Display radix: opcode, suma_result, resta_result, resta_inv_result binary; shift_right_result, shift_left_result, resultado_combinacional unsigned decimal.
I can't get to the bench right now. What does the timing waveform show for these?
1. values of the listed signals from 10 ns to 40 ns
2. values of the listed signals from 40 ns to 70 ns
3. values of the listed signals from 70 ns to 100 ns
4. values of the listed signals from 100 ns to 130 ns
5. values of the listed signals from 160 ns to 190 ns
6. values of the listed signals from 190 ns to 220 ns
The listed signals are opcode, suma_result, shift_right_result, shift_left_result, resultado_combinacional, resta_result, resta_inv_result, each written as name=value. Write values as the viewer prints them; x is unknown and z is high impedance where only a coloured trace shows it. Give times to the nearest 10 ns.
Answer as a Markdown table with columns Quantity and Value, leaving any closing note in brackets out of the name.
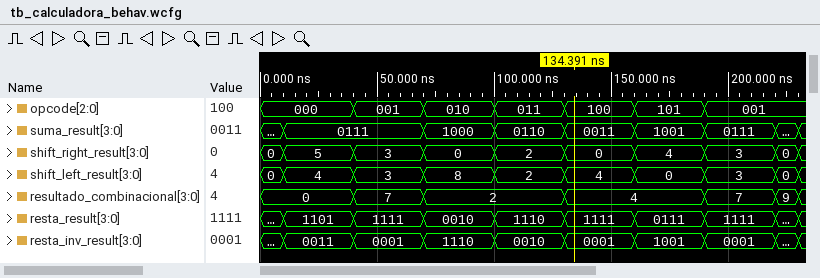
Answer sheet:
| Quantity | Value |
|---|---|
| values of the listed signals from 10 ns to 40 ns | opcode=000, suma_result=0111, shift_right_result=5, shift_left_result=4, resultado_combinacional=0, resta_result=1101, resta_inv_result=0011 |
| values of the listed signals from 40 ns to 70 ns | opcode=001, suma_result=0111, shift_right_result=3, shift_left_result=3, resultado_combinacional=7, resta_result=1111, resta_inv_result=0001 |
| values of the listed signals from 70 ns to 100 ns | opcode=010, suma_result=1000, shift_right_result=0, shift_left_result=8, resultado_combinacional=2, resta_result=0010, resta_inv_result=1110 |
| values of the listed signals from 100 ns to 130 ns | opcode=011, suma_result=0110, shift_right_result=2, shift_left_result=2, resultado_combinacional=2, resta_result=1110, resta_inv_result=0010 |
| values of the listed signals from 160 ns to 190 ns | opcode=101, suma_result=1001, shift_right_result=4, shift_left_result=0, resultado_combinacional=4, resta_result=0111, resta_inv_result=1001 |
| values of the listed signals from 190 ns to 220 ns | opcode=001, suma_result=0111, shift_right_result=3, shift_left_result=3, resultado_combinacional=7, resta_result=1111, resta_inv_result=0001 |
